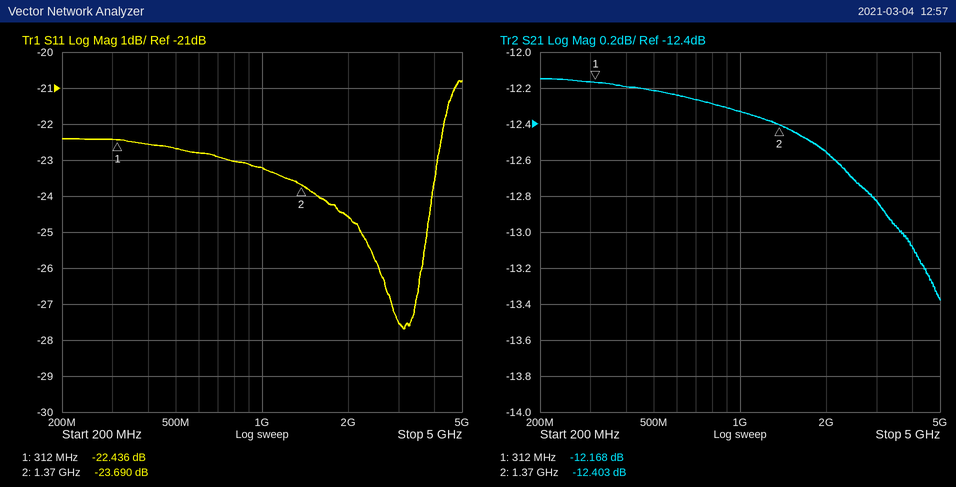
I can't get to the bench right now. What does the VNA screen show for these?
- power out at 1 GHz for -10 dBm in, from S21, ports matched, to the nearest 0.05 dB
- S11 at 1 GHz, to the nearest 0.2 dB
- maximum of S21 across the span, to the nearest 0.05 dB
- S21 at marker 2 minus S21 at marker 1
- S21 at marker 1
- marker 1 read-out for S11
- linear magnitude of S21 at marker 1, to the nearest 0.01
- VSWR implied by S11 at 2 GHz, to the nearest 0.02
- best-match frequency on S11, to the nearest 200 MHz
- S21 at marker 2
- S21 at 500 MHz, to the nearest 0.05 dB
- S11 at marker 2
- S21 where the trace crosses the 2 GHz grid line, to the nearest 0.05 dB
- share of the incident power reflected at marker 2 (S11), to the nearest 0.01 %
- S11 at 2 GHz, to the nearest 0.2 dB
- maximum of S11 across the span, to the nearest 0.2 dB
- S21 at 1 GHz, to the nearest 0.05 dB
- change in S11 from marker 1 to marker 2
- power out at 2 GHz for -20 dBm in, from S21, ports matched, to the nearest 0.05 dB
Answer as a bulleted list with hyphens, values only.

- -22.35 dBm
- -23.2 dB
- -12.15 dB
- -0.235 dB
- -12.168 dB
- -22.436 dB
- 0.25
- 1.12
- 3.2 GHz
- -12.403 dB
- -12.20 dB
- -23.690 dB
- -12.55 dB
- 0.43 %
- -24.6 dB
- -20.8 dB
- -12.35 dB
- -1.254 dB
- -32.55 dBm
